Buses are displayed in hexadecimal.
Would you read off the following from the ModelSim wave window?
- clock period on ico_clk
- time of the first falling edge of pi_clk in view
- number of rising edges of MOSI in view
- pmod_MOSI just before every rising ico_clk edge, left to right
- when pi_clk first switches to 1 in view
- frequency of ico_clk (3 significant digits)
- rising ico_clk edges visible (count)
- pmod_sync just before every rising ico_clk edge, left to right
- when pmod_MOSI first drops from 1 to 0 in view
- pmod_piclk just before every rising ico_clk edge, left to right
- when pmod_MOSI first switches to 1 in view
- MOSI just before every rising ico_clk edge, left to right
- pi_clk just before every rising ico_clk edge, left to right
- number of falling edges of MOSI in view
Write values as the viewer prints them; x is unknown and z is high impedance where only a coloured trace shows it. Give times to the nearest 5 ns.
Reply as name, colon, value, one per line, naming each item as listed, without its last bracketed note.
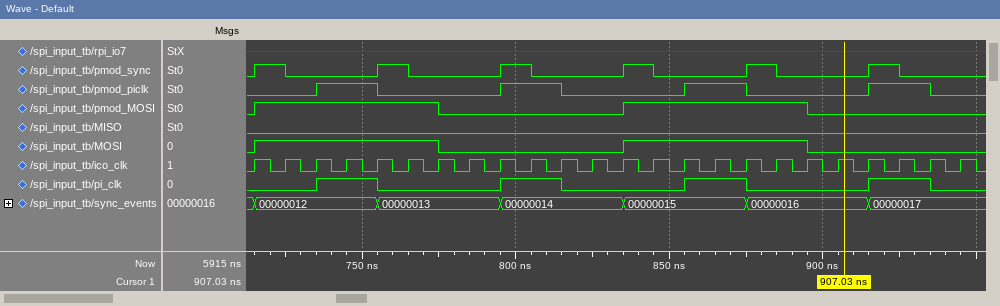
clock period on ico_clk: 10 ns
time of the first falling edge of pi_clk in view: 755 ns
number of rising edges of MOSI in view: 2
pmod_MOSI just before every rising ico_clk edge, left to right: 0 1 1 1 1 1 1 0 0 0 0 0 0 1 1 1 1 1 1 0 0 0 0 0
when pi_clk first switches to 1 in view: 735 ns
frequency of ico_clk: 100 MHz
rising ico_clk edges visible: 24
pmod_sync just before every rising ico_clk edge, left to right: 0 1 0 0 0 1 0 0 0 1 0 0 0 1 0 0 0 1 0 0 0 1 0 0
when pmod_MOSI first drops from 1 to 0 in view: 775 ns
pmod_piclk just before every rising ico_clk edge, left to right: 0 0 0 1 1 0 0 0 0 1 1 0 0 0 0 1 1 0 0 0 0 1 1 0
when pmod_MOSI first switches to 1 in view: 715 ns
MOSI just before every rising ico_clk edge, left to right: 0 1 1 1 1 1 1 0 0 0 0 0 0 1 1 1 1 1 1 0 0 0 0 0
pi_clk just before every rising ico_clk edge, left to right: 0 0 0 1 1 0 0 0 0 1 1 0 0 0 0 1 1 0 0 0 0 1 1 0
number of falling edges of MOSI in view: 2
